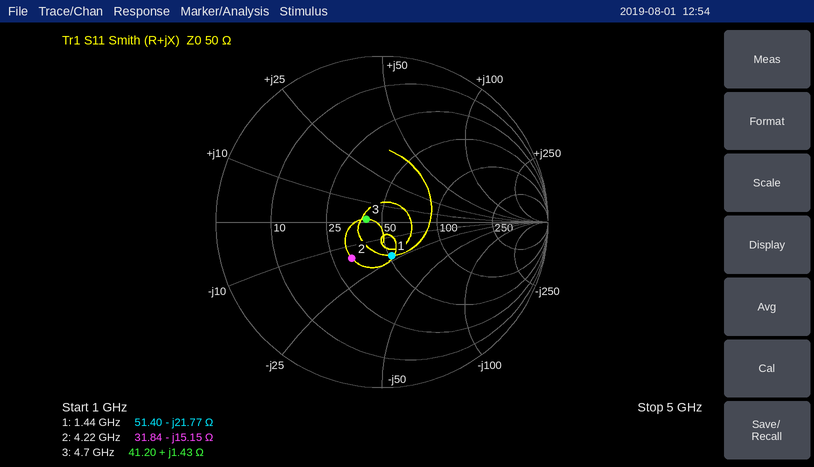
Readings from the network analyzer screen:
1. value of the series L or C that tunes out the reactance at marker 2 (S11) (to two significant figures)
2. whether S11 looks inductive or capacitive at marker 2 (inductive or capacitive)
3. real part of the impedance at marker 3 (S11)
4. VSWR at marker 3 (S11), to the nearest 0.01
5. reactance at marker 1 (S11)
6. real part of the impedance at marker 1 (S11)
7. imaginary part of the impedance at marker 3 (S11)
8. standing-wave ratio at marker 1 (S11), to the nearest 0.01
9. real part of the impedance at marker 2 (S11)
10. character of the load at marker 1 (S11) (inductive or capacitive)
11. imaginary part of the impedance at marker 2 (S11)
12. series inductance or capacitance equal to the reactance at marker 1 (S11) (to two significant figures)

570 pH
capacitive
41.20 Ω
1.22
-21.77 Ω
51.40 Ω
+1.43 Ω
1.53
31.84 Ω
capacitive
-15.15 Ω
5.1 pF
